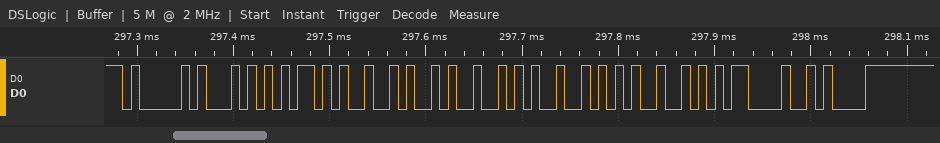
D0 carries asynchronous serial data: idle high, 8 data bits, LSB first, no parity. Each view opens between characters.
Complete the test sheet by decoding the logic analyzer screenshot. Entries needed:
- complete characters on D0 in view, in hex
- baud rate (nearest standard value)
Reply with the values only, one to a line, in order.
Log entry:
41, 54, 2B, 4A, 52, 52, 49, 0D, 0A
115200 baud
